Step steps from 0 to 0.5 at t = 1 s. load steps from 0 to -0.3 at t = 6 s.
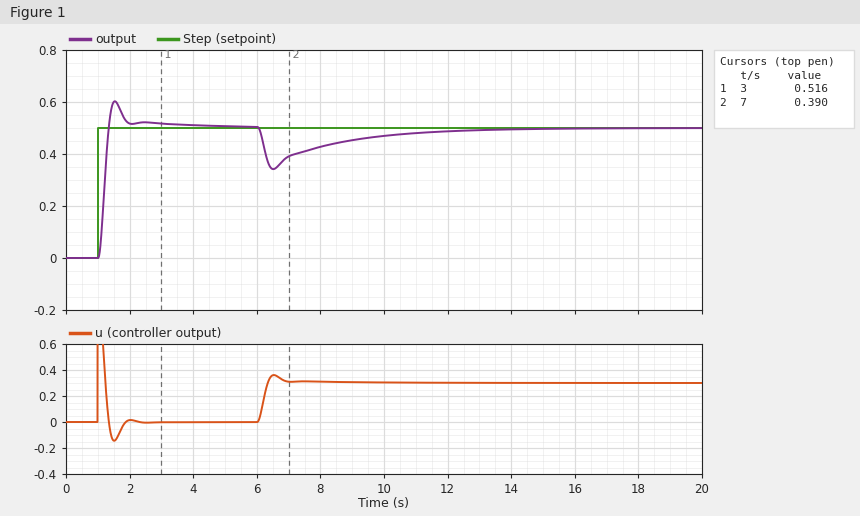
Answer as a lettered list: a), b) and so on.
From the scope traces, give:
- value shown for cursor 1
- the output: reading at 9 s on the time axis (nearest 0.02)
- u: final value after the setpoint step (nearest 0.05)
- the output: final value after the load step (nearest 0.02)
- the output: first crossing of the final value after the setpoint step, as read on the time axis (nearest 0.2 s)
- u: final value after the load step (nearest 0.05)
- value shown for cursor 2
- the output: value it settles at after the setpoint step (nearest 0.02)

a) 0.516
b) 0.46
c) 0.00
d) 0.50
e) 1.4 s
f) 0.30
g) 0.390
h) 0.50
